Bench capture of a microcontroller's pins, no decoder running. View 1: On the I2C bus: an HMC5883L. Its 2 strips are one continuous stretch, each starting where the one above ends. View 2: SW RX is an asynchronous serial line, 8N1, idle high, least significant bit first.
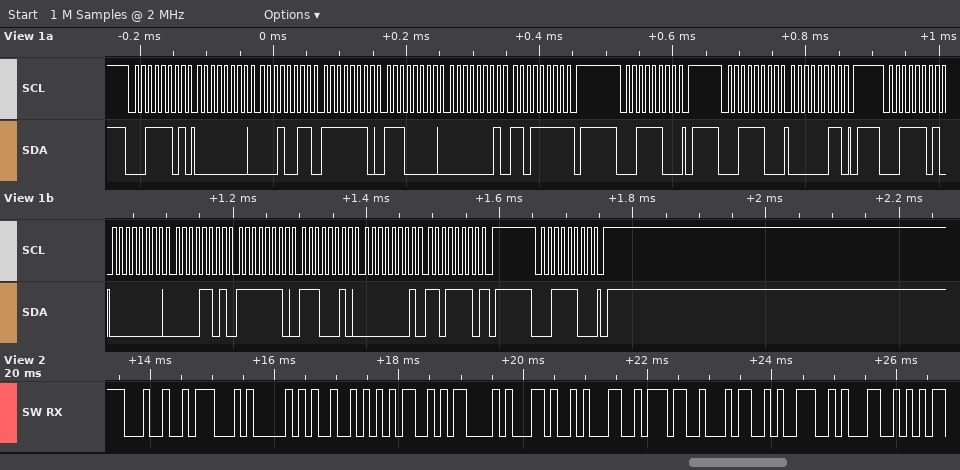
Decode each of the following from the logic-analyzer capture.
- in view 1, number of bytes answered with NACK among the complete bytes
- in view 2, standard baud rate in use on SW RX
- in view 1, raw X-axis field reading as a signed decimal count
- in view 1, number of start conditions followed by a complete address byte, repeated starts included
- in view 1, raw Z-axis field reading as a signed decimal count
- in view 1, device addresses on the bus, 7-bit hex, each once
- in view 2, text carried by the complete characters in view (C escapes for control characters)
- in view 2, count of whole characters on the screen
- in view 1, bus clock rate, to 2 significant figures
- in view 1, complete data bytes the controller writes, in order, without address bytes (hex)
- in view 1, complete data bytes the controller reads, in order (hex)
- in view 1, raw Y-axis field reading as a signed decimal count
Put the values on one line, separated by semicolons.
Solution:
2; 9600 baud; 13; 5; -286; 0x1E; "$GPRMC,17491"; 12; 100 kHz; 03; 00 13 FE E0 01 DF 00 0D FE E2 01 DE; 478
